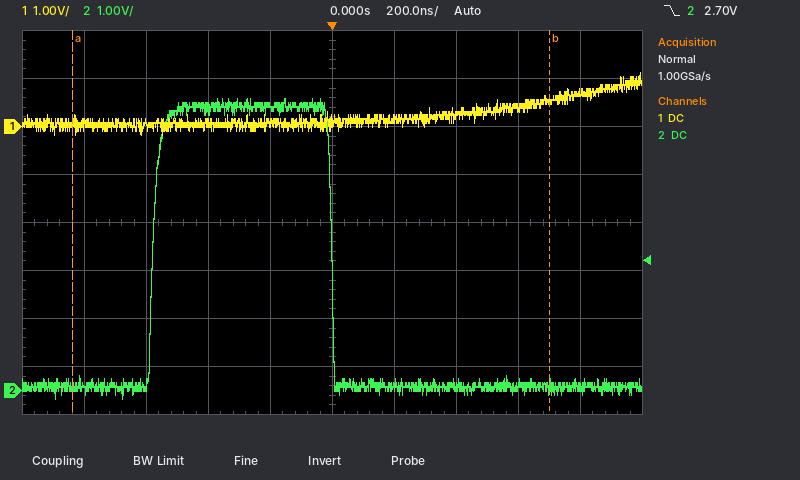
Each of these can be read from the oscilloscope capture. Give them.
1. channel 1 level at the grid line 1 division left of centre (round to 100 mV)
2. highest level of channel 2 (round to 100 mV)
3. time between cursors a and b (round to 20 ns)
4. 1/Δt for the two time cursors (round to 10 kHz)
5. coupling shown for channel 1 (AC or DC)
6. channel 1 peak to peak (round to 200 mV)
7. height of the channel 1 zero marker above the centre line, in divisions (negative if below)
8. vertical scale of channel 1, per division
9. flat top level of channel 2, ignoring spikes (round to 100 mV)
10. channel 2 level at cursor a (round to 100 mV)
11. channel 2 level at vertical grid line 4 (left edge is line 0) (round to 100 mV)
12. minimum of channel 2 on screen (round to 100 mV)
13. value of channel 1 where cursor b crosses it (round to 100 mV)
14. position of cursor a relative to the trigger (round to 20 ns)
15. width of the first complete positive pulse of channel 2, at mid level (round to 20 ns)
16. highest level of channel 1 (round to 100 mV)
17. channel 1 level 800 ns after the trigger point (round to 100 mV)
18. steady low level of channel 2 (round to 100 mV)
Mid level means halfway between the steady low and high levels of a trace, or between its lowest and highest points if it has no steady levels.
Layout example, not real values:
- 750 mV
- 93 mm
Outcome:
- 100 mV
- 6.1 V
- 1.54 µs
- 650 kHz
- DC
- 1.2 V
- +2.0 div
- 1 V
- 5.9 V
- 100 mV
- 5.9 V
- -200 mV
- 500 mV
- -840 ns
- 580 ns
- 1.1 V
- 700 mV
- 100 mV
